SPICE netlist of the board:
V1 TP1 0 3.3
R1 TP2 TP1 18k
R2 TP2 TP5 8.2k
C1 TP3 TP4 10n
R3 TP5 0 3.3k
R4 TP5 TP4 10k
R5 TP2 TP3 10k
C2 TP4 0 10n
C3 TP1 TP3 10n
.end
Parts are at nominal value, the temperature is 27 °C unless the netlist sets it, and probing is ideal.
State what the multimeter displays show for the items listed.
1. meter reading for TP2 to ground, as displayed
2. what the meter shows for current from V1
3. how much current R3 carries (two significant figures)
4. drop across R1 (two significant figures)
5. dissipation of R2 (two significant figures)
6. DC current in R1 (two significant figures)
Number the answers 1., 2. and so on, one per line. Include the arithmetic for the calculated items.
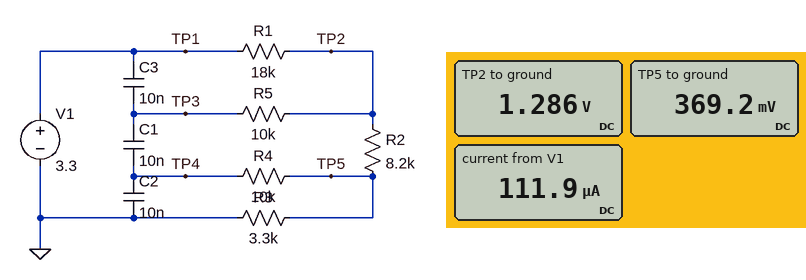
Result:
1. 1.286 V
2. 111.9 µA
3. (369.2 mV) / 3.3 kΩ = 110 µA
4. 3.3 V - 1.286 V = 2.0 V
5. (1.286 V - 369.2 mV)^2 / 8.2 kΩ = 100 µW
6. (3.3 V - 1.286 V) / 18 kΩ = 110 µA
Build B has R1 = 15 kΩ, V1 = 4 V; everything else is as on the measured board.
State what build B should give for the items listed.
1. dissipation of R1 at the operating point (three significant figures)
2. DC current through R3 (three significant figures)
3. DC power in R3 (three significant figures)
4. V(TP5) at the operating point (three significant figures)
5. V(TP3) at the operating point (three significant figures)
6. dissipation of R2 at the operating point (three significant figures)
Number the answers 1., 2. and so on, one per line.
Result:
1. 342 µW
2. 151 µA
3. 75.2 µW
4. 498 mV
5. 1.74 V
6. 187 µW
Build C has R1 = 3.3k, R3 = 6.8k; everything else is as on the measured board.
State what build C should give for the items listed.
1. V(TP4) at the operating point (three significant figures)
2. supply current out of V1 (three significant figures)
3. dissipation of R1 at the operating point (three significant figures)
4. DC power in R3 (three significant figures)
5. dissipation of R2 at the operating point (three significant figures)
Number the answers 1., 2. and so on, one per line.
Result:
1. 1.23 V
2. 180 µA
3. 107 µW
4. 221 µW
5. 267 µW
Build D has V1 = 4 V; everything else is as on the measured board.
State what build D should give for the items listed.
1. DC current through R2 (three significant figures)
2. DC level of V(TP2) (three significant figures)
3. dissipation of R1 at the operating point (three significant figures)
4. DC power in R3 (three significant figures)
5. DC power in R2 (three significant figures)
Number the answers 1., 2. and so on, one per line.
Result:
1. 136 µA
2. 1.56 V
3. 331 µW
4. 60.7 µW
5. 151 µW
